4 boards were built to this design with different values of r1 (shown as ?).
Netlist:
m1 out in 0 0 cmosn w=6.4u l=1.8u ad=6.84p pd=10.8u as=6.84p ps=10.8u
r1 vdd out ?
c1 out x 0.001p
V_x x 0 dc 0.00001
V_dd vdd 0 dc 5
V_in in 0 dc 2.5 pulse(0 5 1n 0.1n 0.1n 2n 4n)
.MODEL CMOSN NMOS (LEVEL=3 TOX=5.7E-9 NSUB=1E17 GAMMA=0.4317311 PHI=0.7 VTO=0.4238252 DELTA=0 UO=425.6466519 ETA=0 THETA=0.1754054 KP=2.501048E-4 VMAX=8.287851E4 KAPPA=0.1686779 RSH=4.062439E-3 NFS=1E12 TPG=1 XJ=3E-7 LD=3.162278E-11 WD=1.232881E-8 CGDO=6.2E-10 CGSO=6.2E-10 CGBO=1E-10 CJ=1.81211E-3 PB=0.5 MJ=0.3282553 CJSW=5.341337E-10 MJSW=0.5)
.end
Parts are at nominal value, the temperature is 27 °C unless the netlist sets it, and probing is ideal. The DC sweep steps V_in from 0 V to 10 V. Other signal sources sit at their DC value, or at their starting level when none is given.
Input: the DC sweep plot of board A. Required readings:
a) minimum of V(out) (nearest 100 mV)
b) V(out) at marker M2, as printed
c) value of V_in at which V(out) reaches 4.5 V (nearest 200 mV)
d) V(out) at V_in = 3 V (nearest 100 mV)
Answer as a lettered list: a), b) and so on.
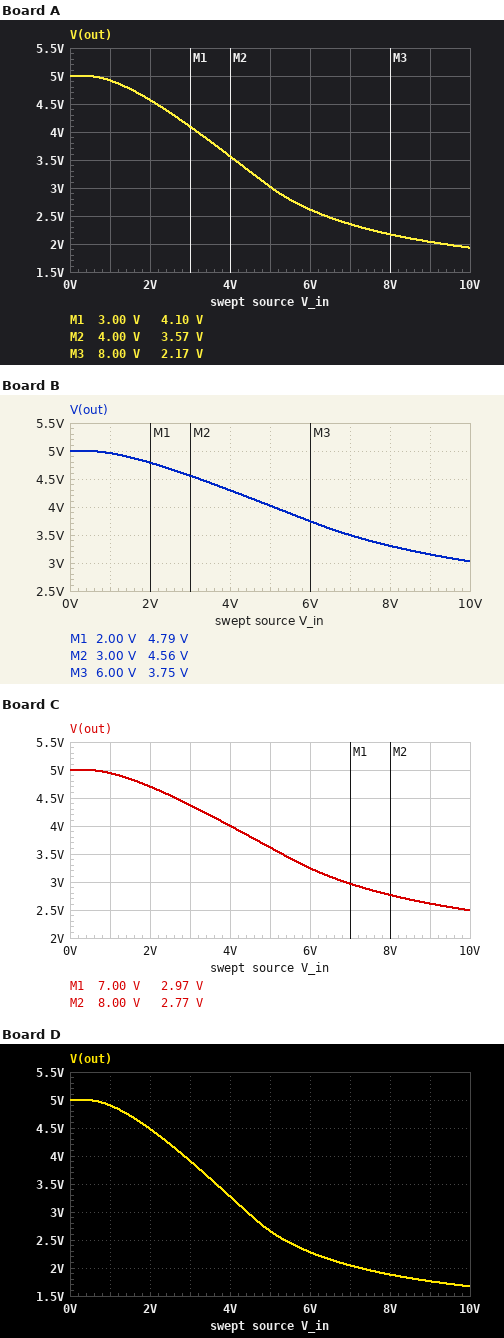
a) 1.9 V
b) 3.57 V
c) 2.2 V
d) 4.1 V
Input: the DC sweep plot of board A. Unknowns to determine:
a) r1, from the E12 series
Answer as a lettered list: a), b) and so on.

a) 680 Ω
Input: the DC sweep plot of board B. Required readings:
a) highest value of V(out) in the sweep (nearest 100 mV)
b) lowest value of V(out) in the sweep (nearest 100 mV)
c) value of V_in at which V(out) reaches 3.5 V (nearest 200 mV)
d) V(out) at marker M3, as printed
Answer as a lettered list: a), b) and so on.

a) 5.0 V
b) 3.0 V
c) 7.0 V
d) 3.75 V
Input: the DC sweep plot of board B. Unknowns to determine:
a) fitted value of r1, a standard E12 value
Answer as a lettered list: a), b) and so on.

a) 330 Ω
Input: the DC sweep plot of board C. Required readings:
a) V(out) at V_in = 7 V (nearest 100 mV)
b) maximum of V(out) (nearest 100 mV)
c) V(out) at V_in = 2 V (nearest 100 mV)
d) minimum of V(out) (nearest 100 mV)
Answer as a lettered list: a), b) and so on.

a) 3.0 V
b) 5.0 V
c) 4.7 V
d) 2.5 V
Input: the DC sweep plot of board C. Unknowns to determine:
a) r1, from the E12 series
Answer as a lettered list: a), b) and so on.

a) 470 Ω
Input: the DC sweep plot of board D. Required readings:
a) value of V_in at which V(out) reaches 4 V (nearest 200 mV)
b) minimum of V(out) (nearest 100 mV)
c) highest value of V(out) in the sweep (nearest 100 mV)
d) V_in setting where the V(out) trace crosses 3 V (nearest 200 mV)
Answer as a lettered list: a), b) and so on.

a) 2.8 V
b) 1.7 V
c) 5.0 V
d) 4.4 V
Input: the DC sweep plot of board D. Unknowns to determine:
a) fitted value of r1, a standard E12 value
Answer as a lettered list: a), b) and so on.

a) 820 Ω
